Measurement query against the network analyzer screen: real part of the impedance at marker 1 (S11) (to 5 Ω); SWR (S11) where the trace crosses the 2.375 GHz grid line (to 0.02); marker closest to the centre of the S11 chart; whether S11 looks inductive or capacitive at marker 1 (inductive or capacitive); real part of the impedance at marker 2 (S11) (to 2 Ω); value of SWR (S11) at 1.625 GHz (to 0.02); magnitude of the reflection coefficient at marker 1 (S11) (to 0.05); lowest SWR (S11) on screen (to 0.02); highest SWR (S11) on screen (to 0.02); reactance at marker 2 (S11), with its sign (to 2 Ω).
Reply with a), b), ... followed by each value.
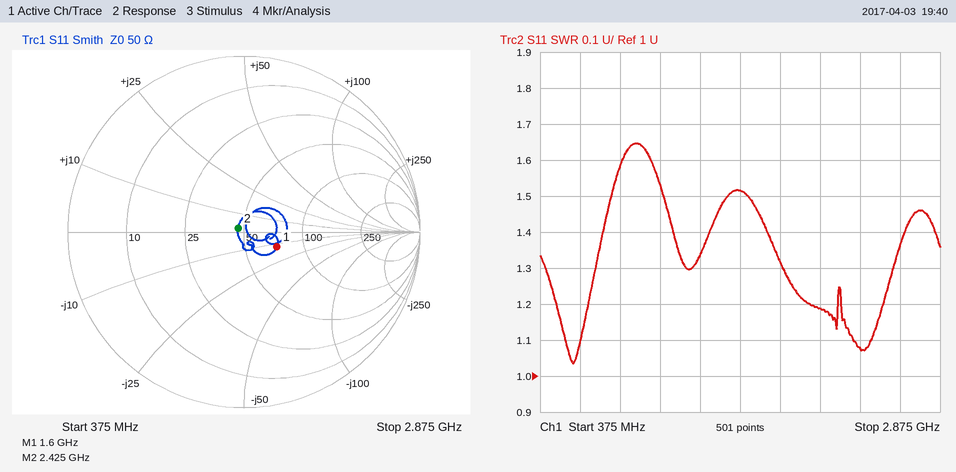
a) 70 Ω
b) 1.08
c) marker 2
d) capacitive
e) 46 Ω
f) 1.52
g) 0.20
h) 1.04
i) 1.64
j) +2 Ω
